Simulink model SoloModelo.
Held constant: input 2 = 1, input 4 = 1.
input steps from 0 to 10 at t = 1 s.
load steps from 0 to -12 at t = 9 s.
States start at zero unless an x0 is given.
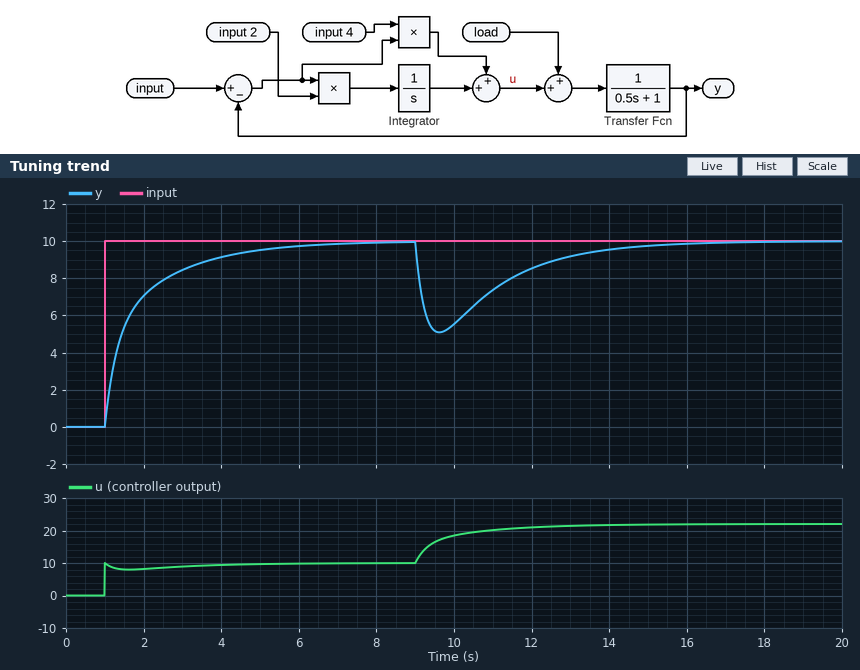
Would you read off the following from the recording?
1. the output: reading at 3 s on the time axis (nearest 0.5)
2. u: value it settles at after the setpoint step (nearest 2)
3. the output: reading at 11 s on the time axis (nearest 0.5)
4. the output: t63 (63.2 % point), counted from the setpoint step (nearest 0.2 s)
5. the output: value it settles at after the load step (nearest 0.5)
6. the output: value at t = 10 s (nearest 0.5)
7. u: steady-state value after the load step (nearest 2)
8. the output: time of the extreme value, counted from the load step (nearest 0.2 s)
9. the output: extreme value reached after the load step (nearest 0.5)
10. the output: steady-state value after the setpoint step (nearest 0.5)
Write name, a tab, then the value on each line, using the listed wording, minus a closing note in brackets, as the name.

the output: reading at 3 s on the time axis	8.5
u: value it settles at after the setpoint step	10
the output: reading at 11 s on the time axis	7.5
the output: t63 (63.2 % point), counted from the setpoint step	0.8 s
the output: value it settles at after the load step	10.0
the output: value at t = 10 s	5.5
u: steady-state value after the load step	22
the output: time of the extreme value, counted from the load step	0.6 s
the output: extreme value reached after the load step	5.0
the output: steady-state value after the setpoint step	10.0
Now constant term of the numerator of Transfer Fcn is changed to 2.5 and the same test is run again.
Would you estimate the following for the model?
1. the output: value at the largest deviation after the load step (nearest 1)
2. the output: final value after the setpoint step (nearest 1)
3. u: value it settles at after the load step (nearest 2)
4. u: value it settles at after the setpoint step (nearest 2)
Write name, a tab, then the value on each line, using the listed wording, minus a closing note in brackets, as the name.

the output: value at the largest deviation after the load step	3
the output: final value after the setpoint step	10
u: value it settles at after the load step	16
u: value it settles at after the setpoint step	4
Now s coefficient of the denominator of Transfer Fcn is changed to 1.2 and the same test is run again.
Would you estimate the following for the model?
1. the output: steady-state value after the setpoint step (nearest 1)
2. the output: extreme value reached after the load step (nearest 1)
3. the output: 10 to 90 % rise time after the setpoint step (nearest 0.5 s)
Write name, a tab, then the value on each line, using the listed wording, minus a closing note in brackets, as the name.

the output: steady-state value after the setpoint step	10
the output: extreme value reached after the load step	6
the output: 10 to 90 % rise time after the setpoint step	2.0 s
